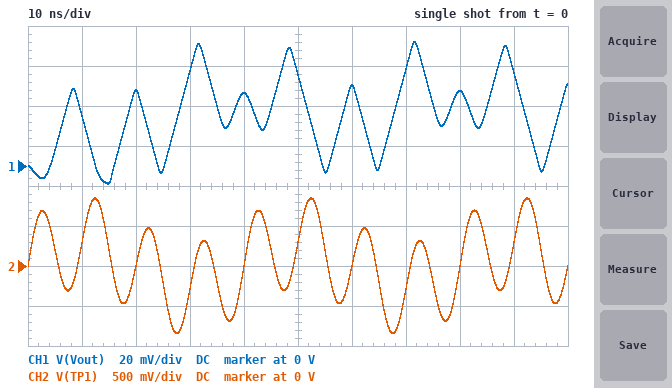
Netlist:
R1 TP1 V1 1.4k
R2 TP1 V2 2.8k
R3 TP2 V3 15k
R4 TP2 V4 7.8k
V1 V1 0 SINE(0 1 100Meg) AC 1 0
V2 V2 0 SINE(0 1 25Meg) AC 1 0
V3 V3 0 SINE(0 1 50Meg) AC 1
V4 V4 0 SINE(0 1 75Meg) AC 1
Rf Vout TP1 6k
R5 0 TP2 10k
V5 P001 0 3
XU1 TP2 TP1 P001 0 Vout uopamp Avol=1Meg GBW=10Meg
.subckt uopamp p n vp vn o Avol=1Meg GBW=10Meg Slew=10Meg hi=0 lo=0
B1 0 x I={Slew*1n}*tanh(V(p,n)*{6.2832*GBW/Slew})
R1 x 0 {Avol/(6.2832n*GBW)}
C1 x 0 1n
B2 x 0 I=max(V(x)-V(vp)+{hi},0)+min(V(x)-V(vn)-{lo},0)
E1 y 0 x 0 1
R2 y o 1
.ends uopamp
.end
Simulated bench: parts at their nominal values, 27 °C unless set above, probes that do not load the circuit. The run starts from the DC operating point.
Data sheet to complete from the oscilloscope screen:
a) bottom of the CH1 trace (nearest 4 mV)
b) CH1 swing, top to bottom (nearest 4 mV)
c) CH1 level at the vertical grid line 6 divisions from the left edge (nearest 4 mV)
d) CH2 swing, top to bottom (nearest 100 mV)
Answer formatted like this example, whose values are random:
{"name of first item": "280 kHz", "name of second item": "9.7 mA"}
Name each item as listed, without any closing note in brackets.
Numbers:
{"bottom of the CH1 trace": "-8 mV", "CH1 swing, top to bottom": "72 mV", "CH1 level at the vertical grid line 6 divisions from the left edge": "40 mV", "CH2 swing, top to bottom": "1.7 V"}
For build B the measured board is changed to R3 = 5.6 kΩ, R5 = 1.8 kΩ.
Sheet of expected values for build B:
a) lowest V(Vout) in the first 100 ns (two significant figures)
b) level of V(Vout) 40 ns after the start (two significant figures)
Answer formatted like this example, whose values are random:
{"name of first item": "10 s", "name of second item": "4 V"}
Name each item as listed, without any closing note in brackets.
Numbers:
{"lowest V(Vout) in the first 100 ns": "-9.2 mV", "level of V(Vout) 40 ns after the start": "60 mV"}
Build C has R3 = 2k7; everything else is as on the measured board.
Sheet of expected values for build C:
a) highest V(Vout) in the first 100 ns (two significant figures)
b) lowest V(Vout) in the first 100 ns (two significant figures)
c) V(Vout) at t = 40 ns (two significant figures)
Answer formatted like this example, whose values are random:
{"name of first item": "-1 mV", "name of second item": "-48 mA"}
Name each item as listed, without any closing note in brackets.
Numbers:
{"highest V(Vout) in the first 100 ns": "68 mV", "lowest V(Vout) in the first 100 ns": "-7.5 mV", "V(Vout) at t = 40 ns": "23 mV"}
